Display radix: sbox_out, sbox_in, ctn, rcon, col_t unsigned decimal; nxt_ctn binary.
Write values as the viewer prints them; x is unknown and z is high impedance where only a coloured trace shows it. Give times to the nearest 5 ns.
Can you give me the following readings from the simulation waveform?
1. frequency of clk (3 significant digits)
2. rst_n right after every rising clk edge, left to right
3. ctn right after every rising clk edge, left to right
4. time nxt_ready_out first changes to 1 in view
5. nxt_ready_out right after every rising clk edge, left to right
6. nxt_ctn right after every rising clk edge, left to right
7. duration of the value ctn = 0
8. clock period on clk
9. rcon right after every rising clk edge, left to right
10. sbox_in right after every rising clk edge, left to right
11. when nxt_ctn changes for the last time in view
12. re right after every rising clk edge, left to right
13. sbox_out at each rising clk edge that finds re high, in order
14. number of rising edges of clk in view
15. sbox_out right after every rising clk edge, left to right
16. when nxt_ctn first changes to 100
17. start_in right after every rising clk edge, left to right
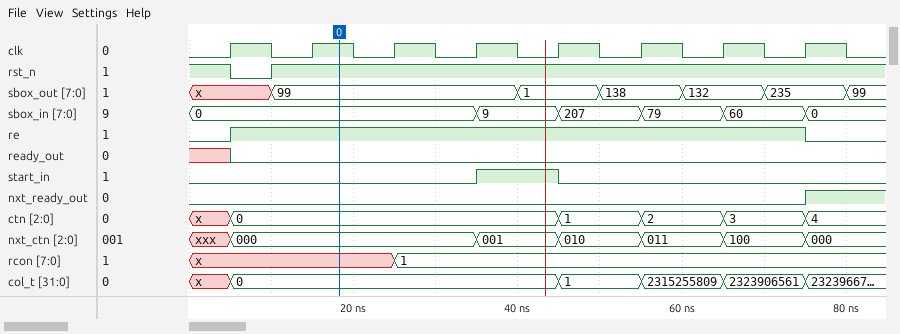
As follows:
100 MHz
0 1 1 1 1 1 1 1
0, 0, 0, 0, 1, 2, 3, 4
75 ns
0 0 0 0 0 0 0 1
000, 000, 000, 001, 010, 011, 100, 000
40 ns
10 ns
x, x, 1, 1, 1, 1, 1, 1
0, 0, 0, 9, 207, 79, 60, 0
75 ns
1 1 1 1 1 1 1 0
99, 99, 99, 1, 138, 132, 235
8
x, 99, 99, 99, 1, 138, 132, 235
65 ns
0 0 0 1 0 0 0 0
